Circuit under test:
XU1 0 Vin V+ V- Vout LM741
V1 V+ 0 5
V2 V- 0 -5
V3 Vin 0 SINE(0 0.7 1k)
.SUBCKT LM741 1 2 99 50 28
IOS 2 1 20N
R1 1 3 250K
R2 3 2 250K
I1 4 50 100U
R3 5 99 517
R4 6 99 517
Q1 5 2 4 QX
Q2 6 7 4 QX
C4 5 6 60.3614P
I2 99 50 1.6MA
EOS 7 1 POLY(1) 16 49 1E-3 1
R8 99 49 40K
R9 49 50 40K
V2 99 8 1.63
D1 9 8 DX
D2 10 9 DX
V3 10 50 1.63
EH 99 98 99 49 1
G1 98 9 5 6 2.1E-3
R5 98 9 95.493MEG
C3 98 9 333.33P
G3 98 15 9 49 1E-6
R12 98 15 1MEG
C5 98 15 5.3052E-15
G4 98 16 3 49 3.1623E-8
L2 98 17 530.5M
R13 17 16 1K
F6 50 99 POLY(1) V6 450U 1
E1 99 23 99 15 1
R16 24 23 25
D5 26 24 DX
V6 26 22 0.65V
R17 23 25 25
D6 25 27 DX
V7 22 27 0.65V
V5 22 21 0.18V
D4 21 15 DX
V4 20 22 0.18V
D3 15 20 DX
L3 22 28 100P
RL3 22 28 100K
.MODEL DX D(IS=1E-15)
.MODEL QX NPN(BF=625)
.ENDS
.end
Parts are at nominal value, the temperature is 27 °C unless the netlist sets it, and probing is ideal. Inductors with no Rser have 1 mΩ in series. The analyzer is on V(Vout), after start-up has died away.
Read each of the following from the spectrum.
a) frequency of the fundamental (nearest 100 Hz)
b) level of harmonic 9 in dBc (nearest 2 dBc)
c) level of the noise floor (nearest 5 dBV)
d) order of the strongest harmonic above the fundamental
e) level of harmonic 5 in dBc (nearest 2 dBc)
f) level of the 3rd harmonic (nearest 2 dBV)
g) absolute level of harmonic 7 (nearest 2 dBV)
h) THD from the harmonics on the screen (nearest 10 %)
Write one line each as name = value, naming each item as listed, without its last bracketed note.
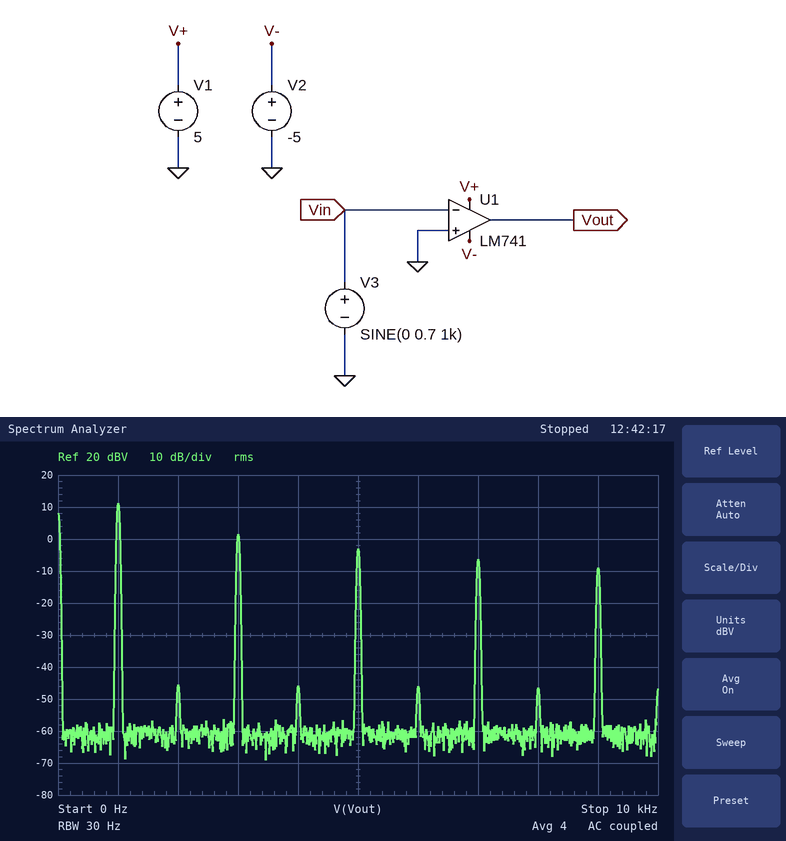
frequency of the fundamental = 1.0 kHz
level of harmonic 9 in dBc = -20 dBc
level of the noise floor = -60 dBV
order of the strongest harmonic above the fundamental = 3
level of harmonic 5 in dBc = -14 dBc
level of the 3rd harmonic = 2 dBV
absolute level of harmonic 7 = -6 dBV
THD from the harmonics on the screen = 40 %
